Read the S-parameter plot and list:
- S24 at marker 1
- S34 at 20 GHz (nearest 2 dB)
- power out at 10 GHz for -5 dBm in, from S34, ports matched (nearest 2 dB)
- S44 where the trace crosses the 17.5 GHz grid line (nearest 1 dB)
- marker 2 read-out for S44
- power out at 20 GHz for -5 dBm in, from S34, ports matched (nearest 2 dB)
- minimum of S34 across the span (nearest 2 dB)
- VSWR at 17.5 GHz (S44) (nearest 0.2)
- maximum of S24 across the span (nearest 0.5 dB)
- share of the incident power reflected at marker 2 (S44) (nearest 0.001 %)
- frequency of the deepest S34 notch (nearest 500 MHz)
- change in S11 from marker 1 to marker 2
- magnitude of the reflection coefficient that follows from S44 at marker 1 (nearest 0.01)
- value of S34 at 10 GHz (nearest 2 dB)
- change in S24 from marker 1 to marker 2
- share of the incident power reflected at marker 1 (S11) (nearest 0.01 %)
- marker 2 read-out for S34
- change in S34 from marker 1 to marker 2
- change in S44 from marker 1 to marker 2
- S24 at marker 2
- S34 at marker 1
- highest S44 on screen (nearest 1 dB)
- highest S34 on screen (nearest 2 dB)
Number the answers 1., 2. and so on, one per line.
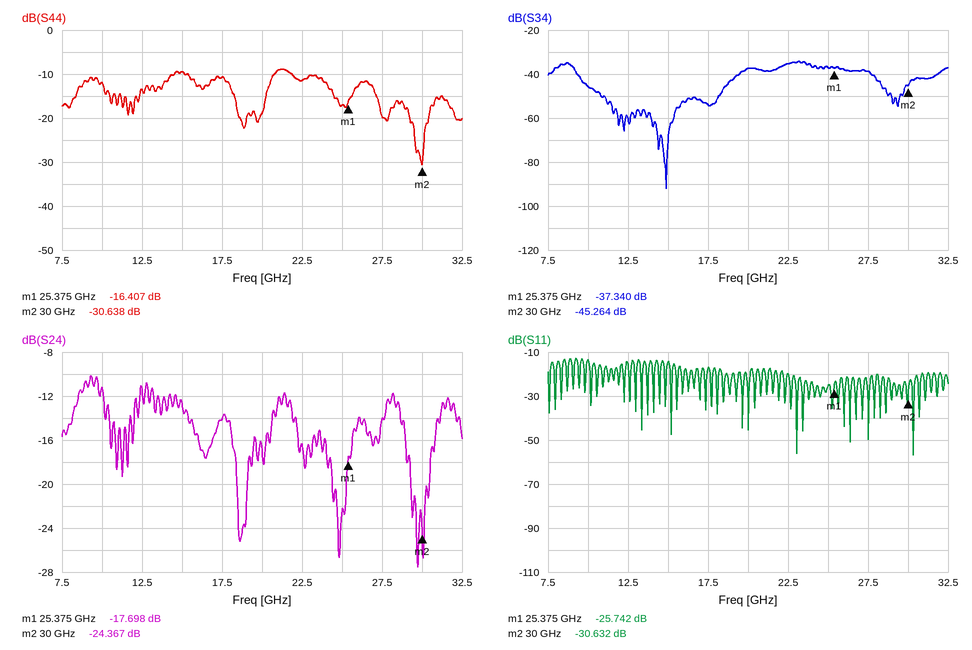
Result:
1. -17.698 dB
2. -38 dB
3. -50 dBm
4. -11 dB
5. -30.638 dB
6. -42 dBm
7. -92 dB
8. 1.8
9. -10.0 dB
10. 0.086 %
11. 15.0 GHz
12. -4.890 dB
13. 0.15
14. -46 dB
15. -6.669 dB
16. 0.27 %
17. -45.264 dB
18. -7.924 dB
19. -14.231 dB
20. -24.367 dB
21. -37.340 dB
22. -9 dB
23. -34 dB
